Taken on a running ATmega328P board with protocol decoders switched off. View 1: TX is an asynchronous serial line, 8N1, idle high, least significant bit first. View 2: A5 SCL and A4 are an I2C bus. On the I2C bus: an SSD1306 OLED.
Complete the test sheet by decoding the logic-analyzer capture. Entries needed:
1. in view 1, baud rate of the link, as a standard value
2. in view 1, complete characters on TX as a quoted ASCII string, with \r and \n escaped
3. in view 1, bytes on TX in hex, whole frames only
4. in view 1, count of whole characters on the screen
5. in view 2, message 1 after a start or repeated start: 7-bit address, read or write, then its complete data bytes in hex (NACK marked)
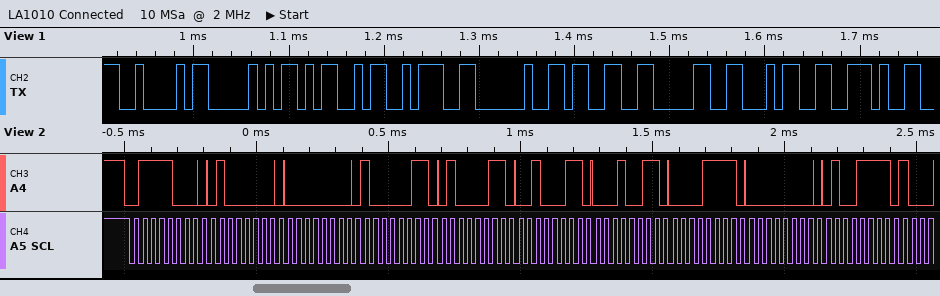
115200 baud
"BPM: 304."
42 50 4D 3A 20 33 30 34 2E
9
0x3C write: 40 00 83 43 23 13 0F 00 4F
